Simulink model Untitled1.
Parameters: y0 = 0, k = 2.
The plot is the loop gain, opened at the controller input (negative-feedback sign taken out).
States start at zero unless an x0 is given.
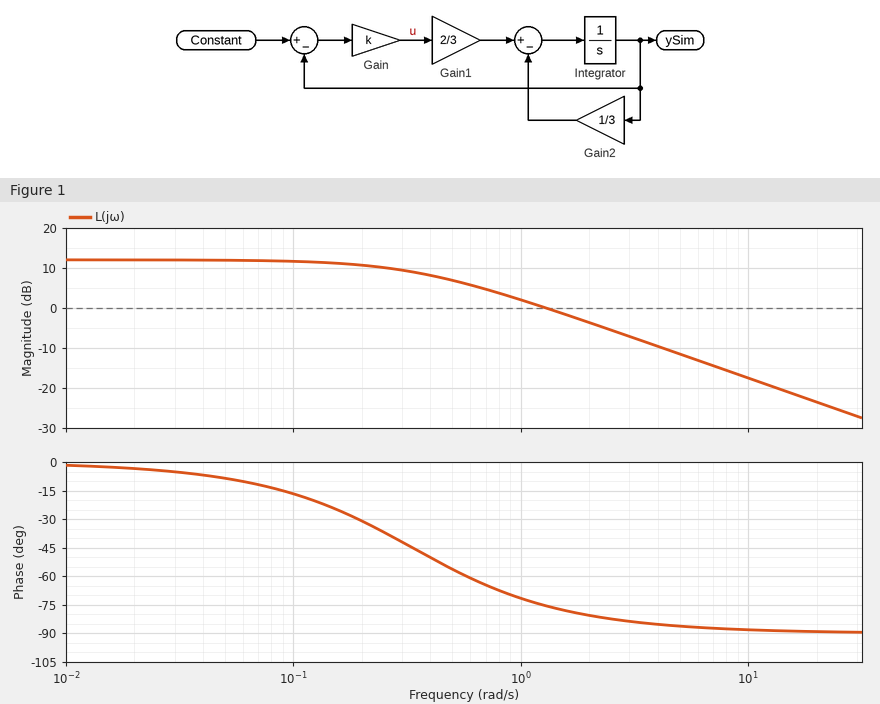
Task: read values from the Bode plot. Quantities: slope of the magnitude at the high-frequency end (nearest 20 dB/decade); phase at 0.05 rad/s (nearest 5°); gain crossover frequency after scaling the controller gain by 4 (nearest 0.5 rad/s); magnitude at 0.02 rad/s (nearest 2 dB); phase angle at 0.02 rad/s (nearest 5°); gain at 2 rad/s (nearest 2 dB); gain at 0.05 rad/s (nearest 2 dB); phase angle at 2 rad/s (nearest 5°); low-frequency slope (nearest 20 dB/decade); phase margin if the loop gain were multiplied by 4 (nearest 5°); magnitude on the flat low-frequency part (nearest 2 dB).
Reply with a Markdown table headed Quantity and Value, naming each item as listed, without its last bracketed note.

| Quantity | Value |
|---|---|
| slope of the magnitude at the high-frequency end | -20 dB/decade |
| phase at 0.05 rad/s | -10° |
| gain crossover frequency after scaling the controller gain by 4 | 5.5 rad/s |
| magnitude at 0.02 rad/s | 12 dB |
| phase angle at 0.02 rad/s | -5° |
| gain at 2 rad/s | -4 dB |
| gain at 0.05 rad/s | 12 dB |
| phase angle at 2 rad/s | -80° |
| low-frequency slope | 0 dB/decade |
| phase margin if the loop gain were multiplied by 4 | 95° |
| magnitude on the flat low-frequency part | 12 dB |
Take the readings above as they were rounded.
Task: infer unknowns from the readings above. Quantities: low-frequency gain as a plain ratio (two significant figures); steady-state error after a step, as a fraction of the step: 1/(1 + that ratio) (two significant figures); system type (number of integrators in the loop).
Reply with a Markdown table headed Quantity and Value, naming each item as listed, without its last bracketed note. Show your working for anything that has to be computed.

| Quantity | Value |
|---|---|
| low-frequency gain as a plain ratio | 10^(12 / 20) = 4.0 |
| steady-state error after a step, as a fraction of the step: 1/(1 + that ratio) | 1 / (1 + 4) = 0.20 |
| system type | 0 |
